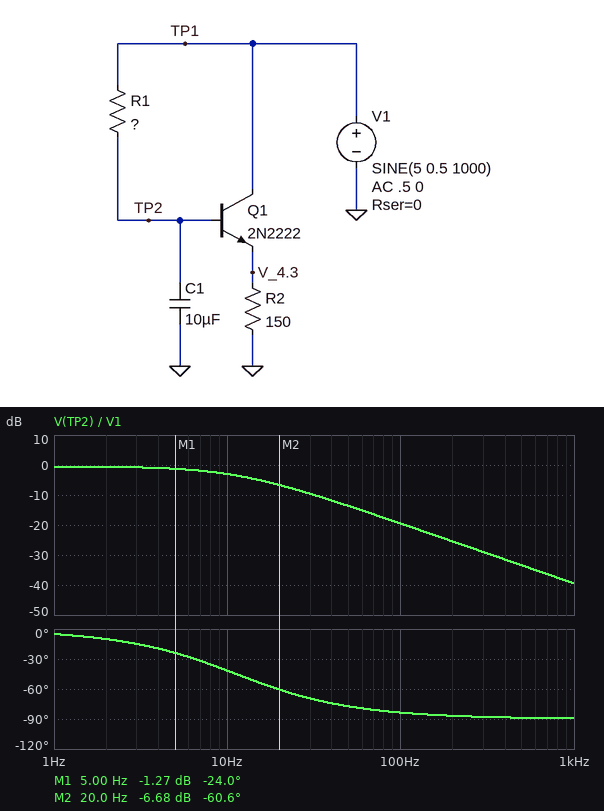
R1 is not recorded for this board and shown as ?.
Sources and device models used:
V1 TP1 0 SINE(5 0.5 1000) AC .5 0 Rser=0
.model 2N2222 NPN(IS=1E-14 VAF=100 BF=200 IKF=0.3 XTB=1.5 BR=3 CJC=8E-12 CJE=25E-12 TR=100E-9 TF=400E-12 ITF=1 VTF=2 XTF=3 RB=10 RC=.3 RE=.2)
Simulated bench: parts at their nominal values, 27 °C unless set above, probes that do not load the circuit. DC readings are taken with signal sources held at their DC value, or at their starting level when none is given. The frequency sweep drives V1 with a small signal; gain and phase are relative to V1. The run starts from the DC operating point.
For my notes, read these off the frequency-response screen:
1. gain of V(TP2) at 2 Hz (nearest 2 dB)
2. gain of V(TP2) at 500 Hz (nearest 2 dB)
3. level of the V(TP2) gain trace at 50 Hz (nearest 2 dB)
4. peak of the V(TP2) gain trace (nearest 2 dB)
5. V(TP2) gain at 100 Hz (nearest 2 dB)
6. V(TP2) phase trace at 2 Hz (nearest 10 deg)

0 dB
-34 dB
-14 dB
0 dB
-20 dB
-10 deg
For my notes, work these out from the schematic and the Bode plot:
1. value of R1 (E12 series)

1.5 kΩ
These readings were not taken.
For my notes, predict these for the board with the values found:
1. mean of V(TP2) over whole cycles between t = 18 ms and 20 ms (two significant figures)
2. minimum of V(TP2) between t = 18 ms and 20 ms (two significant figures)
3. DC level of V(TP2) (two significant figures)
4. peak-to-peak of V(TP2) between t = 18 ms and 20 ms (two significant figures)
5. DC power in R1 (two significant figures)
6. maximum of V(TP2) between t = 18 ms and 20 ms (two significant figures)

4.8 V
4.8 V
4.8 V
11 mV
32 µW
4.8 V
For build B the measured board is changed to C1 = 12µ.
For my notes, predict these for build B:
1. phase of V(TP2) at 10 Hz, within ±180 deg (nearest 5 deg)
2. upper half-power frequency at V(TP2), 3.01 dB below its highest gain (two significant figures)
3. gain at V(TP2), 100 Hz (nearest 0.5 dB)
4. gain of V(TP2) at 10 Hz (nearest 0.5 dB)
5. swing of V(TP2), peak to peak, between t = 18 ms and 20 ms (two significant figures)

-45 deg
9.4 Hz
-21.0 dB
-4.0 dB
9.0 mV
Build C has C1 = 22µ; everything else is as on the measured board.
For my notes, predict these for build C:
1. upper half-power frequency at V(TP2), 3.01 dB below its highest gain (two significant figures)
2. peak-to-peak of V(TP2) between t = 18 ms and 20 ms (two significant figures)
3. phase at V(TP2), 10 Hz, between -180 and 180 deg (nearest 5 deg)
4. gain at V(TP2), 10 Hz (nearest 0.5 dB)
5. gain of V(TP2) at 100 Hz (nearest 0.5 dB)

5.1 Hz
4.9 mV
-65 deg
-7.5 dB
-26.5 dB
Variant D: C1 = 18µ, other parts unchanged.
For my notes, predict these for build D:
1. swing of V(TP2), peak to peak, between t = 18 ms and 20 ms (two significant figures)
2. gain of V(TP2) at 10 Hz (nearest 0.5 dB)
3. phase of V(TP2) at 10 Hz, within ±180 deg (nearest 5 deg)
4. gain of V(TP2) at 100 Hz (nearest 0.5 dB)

6.0 mV
-6.0 dB
-60 deg
-24.5 dB
